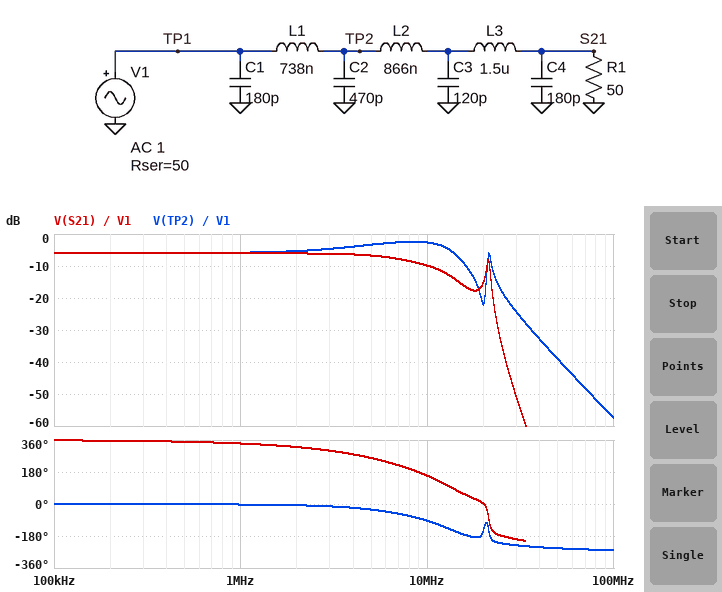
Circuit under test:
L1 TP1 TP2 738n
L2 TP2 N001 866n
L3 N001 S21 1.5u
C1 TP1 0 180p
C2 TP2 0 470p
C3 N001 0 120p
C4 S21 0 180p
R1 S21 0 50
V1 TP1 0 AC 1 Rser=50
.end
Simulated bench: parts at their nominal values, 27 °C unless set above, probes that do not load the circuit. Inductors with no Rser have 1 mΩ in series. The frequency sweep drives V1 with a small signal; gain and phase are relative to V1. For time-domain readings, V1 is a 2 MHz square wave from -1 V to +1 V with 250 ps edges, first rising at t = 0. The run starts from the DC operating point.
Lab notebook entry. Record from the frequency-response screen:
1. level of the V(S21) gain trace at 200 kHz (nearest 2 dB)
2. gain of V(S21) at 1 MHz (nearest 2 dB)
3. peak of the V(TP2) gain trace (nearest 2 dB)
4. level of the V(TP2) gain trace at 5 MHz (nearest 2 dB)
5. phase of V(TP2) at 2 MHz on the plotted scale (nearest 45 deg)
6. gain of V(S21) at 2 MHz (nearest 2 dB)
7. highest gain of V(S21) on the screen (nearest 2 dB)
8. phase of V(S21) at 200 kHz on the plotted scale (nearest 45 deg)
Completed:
-6 dB
-6 dB
-2 dB
-4 dB
0 deg
-6 dB
-6 dB
360 deg
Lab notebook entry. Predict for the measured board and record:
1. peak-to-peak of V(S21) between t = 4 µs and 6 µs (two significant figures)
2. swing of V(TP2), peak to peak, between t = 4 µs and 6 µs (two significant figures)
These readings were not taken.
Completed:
1.1 V
1.8 V
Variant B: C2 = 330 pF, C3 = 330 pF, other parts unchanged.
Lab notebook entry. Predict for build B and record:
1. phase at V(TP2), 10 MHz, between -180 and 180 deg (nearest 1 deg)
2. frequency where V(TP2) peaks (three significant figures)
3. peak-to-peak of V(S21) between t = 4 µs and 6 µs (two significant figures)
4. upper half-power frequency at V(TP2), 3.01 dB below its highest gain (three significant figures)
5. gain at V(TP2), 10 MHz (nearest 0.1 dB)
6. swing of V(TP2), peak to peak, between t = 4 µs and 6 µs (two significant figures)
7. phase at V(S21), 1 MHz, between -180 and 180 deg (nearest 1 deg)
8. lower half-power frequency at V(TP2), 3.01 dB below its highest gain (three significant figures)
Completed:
-89 deg
16.8 MHz
1.2 V
18.2 MHz
-6.6 dB
1.6 V
-20 deg
15.4 MHz
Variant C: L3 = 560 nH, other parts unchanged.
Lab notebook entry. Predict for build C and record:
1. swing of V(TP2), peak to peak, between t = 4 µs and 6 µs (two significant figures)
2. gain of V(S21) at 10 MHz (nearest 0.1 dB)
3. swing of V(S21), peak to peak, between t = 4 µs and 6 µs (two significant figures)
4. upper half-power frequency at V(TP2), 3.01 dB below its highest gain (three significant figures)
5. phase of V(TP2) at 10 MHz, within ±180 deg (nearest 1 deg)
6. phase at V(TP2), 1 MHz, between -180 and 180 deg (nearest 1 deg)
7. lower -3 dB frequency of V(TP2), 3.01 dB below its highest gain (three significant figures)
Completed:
1.6 V
-6.9 dB
1.2 V
15.6 MHz
-76 deg
-6 deg
3.53 MHz
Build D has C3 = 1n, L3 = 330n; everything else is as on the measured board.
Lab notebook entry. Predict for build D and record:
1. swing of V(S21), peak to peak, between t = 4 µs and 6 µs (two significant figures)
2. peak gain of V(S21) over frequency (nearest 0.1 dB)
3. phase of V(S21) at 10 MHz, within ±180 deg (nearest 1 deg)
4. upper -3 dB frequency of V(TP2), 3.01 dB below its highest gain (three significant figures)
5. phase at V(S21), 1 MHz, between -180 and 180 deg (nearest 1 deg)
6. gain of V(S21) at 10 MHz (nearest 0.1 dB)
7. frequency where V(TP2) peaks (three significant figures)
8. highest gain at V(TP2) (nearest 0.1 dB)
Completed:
1.0 V
-6.0 dB
136 deg
15.3 MHz
-23 deg
-9.3 dB
12.5 MHz
0.3 dB
